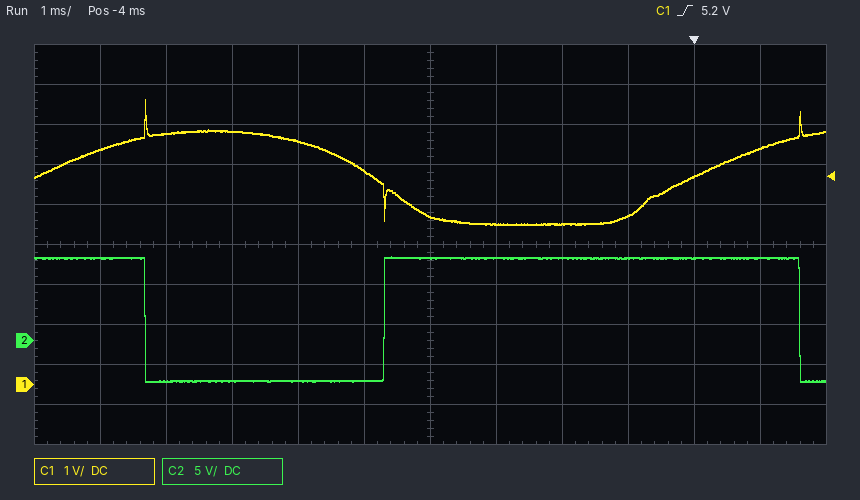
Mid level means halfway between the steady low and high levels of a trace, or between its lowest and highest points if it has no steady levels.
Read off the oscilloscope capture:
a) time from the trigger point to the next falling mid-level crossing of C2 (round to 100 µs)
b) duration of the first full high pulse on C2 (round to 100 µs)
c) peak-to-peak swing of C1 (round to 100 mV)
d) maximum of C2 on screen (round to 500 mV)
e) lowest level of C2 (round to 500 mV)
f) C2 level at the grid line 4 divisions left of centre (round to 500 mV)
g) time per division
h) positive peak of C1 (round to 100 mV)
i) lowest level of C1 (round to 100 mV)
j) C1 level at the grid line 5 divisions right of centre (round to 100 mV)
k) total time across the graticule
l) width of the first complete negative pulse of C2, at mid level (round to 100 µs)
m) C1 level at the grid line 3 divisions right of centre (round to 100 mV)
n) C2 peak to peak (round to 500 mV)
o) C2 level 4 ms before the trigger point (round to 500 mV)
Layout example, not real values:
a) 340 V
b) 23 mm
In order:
a) 1.6 ms
b) 6.3 ms
c) 3.1 V
d) 10.5 V
e) -5.0 V
f) -5.0 V
g) 1 ms
h) 7.1 V
i) 4.0 V
j) 5.9 V
k) 12 ms
l) 3.6 ms
m) 4.2 V
n) 15.5 V
o) 10.5 V
